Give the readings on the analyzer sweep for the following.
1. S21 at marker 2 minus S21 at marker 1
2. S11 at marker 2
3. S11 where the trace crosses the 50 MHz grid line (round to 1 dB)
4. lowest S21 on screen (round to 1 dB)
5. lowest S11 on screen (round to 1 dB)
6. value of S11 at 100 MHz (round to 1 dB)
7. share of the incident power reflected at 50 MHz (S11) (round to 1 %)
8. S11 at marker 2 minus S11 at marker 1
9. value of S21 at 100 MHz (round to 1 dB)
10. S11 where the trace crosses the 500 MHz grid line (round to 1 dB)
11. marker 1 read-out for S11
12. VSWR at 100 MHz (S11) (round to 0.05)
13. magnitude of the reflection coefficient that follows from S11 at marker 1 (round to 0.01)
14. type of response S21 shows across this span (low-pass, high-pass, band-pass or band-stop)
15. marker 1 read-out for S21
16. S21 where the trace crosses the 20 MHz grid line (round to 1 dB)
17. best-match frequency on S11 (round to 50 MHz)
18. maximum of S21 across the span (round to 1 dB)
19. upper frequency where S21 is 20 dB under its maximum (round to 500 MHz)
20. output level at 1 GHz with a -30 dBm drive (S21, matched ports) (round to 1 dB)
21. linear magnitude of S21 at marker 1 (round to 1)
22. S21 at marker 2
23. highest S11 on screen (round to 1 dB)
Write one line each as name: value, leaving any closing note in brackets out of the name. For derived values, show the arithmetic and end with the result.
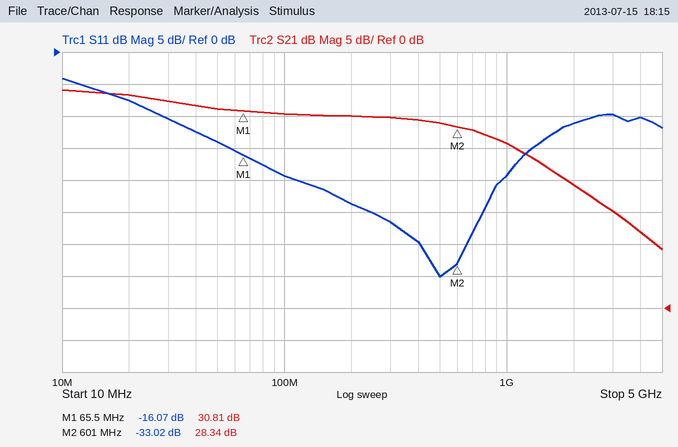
S21 at marker 2 minus S21 at marker 1: 28.34 − (30.81) = -2.47 dB
S11 at marker 2: -33.02 dB
S11 where the trace crosses the 50 MHz grid line: -14 dB
lowest S21 on screen: 9 dB
lowest S11 on screen: -35 dB
value of S11 at 100 MHz: -19 dB
share of the incident power reflected at 50 MHz (S11): 10^(-14/10) ≈ 4 %
S11 at marker 2 minus S11 at marker 1: -33.02 − (-16.07) = -16.95 dB
value of S21 at 100 MHz: 30 dB
S11 where the trace crosses the 500 MHz grid line: -35 dB
marker 1 read-out for S11: -16.07 dB
VSWR at 100 MHz (S11): |Γ| = 10^(-19/20) = 0.1122; VSWR = (1 + 0.1122)/(1 − 0.1122) ≈ 1.25
magnitude of the reflection coefficient that follows from S11 at marker 1: 10^(-16.07/20) ≈ 0.16
type of response S21 shows across this span: low-pass
marker 1 read-out for S21: 30.81 dB
S21 where the trace crosses the 20 MHz grid line: 33 dB
best-match frequency on S11: 500 MHz
maximum of S21 across the span: 34 dB
upper frequency where S21 is 20 dB under its maximum: 3.5 GHz
output level at 1 GHz with a -30 dBm drive (S21, matched ports): -30 dBm + (26 dB) = -4 dBm
linear magnitude of S21 at marker 1: 10^(30.81/20) ≈ 35
S21 at marker 2: 28.34 dB
highest S11 on screen: -4 dB
